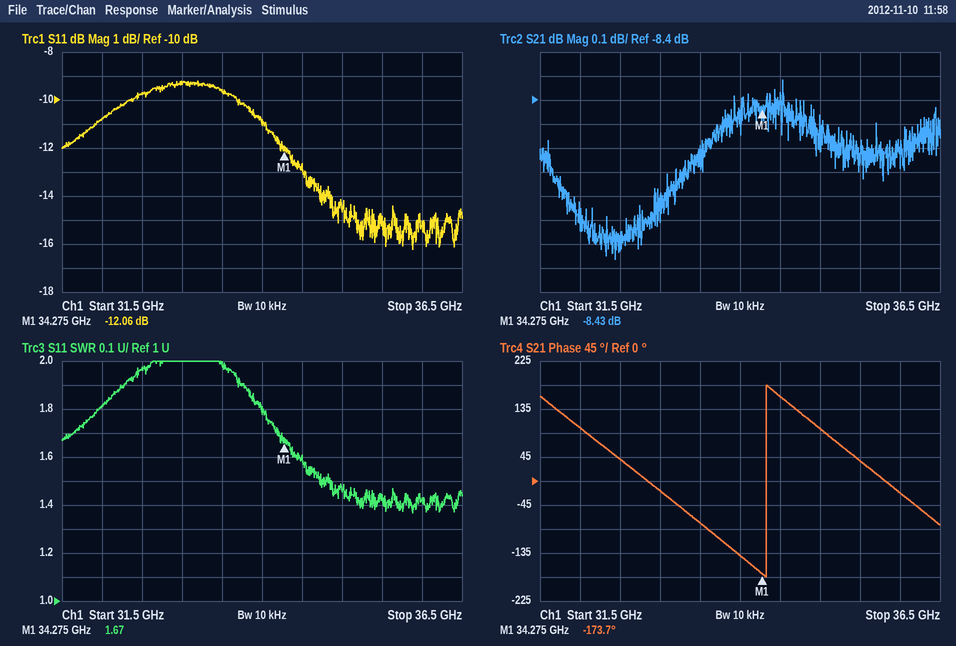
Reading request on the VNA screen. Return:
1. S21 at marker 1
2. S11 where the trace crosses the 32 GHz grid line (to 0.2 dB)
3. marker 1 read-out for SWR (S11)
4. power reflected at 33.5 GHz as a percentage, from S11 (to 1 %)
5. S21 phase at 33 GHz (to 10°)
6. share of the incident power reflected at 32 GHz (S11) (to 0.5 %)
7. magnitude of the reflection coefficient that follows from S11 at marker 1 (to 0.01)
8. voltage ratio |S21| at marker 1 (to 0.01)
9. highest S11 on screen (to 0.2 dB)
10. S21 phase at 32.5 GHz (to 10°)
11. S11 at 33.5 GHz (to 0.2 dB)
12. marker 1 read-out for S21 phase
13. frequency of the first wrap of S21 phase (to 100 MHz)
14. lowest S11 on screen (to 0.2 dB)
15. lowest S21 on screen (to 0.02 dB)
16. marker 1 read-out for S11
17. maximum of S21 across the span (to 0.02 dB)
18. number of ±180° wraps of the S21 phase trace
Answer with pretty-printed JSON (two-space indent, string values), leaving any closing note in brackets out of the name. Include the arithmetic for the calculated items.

{
  "S21 at marker 1": "-8.43 dB",
  "S11 where the trace crosses the 32 GHz grid line": "-10.8 dB",
  "marker 1 read-out for SWR": "1.67",
  "power reflected at 33.5 GHz as a percentage, from S11": "10^(-9.6/10) ≈ 11 %",
  "S21 phase at 33 GHz": "-20°",
  "share of the incident power reflected at 32 GHz (S11)": "10^(-10.8/10) ≈ 8.32 %, so 8.5 % to the nearest 0.5 %",
  "magnitude of the reflection coefficient that follows from S11 at marker 1": "10^(-12.06/20) ≈ 0.25",
  "voltage ratio |S21| at marker 1": "10^(-8.43/20) ≈ 0.38",
  "highest S11 on screen": "-9.2 dB",
  "S21 phase at 32.5 GHz": "40°",
  "S11 at 33.5 GHz": "-9.6 dB",
  "marker 1 read-out for S21 phase": "-173.7°",
  "frequency of the first wrap of S21 phase": "34.3 GHz",
  "lowest S11 on screen": "-16.2 dB",
  "lowest S21 on screen": "-9.06 dB",
  "marker 1 read-out for S11": "-12.06 dB",
  "maximum of S21 across the span": "-8.32 dB",
  "number of ±180° wraps of the S21 phase trace": "1"
}
